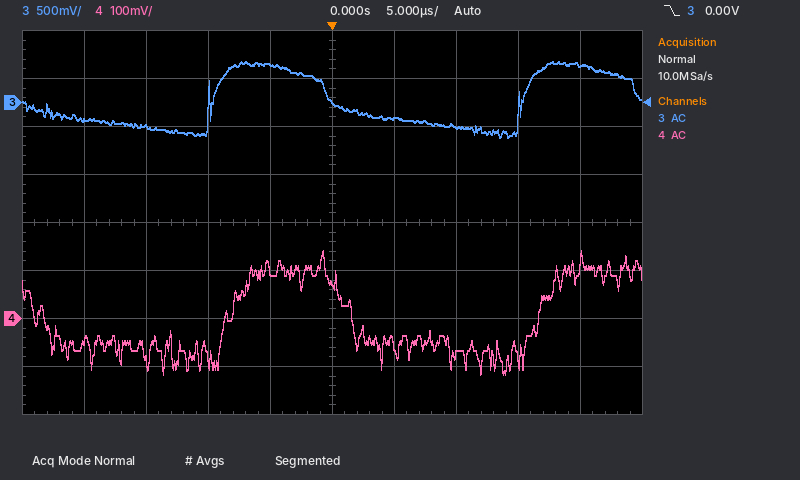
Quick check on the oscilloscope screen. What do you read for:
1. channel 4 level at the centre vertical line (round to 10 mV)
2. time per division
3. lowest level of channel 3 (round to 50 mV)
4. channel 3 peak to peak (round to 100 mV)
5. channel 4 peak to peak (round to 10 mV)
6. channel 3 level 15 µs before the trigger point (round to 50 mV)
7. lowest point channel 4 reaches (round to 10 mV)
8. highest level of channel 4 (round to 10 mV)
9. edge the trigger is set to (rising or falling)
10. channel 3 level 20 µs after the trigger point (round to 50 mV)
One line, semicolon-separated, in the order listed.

70 mV; 5 µs; -350 mV; 800 mV; 260 mV; -250 mV; -120 mV; 140 mV; falling; 400 mV
